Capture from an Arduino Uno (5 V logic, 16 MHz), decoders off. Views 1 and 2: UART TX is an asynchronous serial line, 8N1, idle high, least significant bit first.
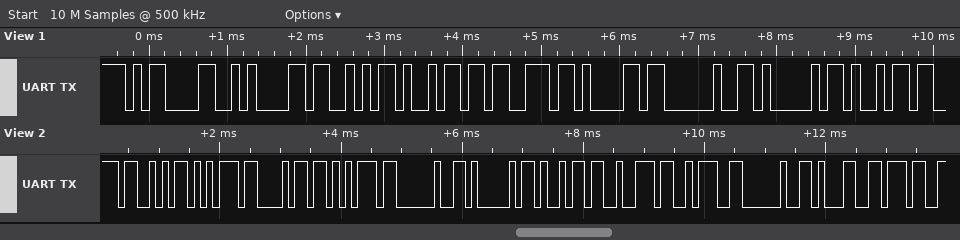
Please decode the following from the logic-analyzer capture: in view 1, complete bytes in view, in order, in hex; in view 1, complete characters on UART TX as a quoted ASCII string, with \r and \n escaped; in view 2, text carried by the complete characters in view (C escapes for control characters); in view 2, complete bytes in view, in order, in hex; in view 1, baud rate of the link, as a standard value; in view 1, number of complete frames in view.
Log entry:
0D 0A 53 69 73 61 20 41 69
"\r\nSisa Ai"
"Suhu Air: 17"
53 75 68 75 20 41 69 72 3A 20 31 37
9600 baud
9
